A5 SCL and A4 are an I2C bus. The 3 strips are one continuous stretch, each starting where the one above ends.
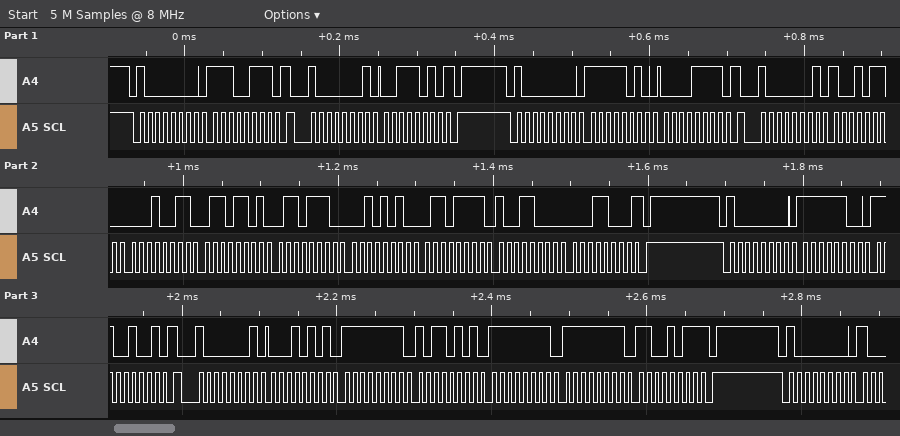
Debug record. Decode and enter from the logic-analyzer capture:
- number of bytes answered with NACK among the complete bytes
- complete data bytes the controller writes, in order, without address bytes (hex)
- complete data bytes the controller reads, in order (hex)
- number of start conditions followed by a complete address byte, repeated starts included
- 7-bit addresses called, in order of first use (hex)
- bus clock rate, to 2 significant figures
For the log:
3
E7 FA 0F FC C9
3A 96 13 6D 6E 2A 6F 98 18 15 FF B5 FF FF CB
7
0x40
100 kHz
